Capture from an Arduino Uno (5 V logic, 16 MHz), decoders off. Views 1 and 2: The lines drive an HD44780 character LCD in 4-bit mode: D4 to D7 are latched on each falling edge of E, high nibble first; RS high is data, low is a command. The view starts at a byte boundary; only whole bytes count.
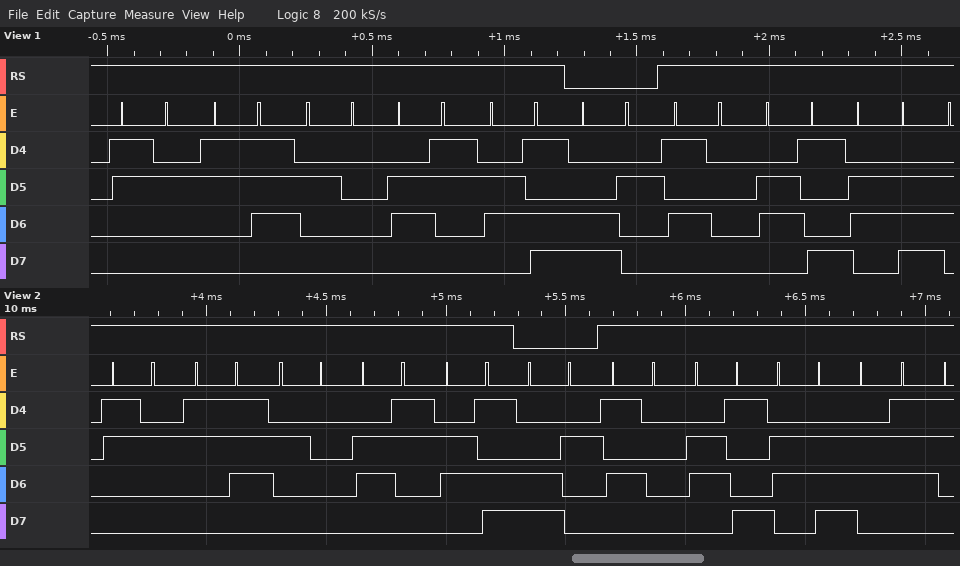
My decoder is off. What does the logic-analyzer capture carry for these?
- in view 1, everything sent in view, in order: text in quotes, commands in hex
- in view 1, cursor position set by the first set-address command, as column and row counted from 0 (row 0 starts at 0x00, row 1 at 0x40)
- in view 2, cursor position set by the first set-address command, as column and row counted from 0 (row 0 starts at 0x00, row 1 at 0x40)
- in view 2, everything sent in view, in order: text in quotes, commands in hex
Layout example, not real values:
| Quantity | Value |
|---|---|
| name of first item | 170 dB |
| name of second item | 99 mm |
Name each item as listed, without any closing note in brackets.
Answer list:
| Quantity | Value |
|---|---|
| in view 1, everything sent in view, in order: text in quotes, commands in hex | "27 cm" 0xC2 "Pin" |
| in view 1, cursor position set by the first set-address command, as column and row counted from 0 | column 2, row 1 |
| in view 2, cursor position set by the first set-address command, as column and row counted from 0 | column 2, row 1 |
| in view 2, everything sent in view, in order: text in quotes, commands in hex | "27 cm" 0xC2 "Ping" |
